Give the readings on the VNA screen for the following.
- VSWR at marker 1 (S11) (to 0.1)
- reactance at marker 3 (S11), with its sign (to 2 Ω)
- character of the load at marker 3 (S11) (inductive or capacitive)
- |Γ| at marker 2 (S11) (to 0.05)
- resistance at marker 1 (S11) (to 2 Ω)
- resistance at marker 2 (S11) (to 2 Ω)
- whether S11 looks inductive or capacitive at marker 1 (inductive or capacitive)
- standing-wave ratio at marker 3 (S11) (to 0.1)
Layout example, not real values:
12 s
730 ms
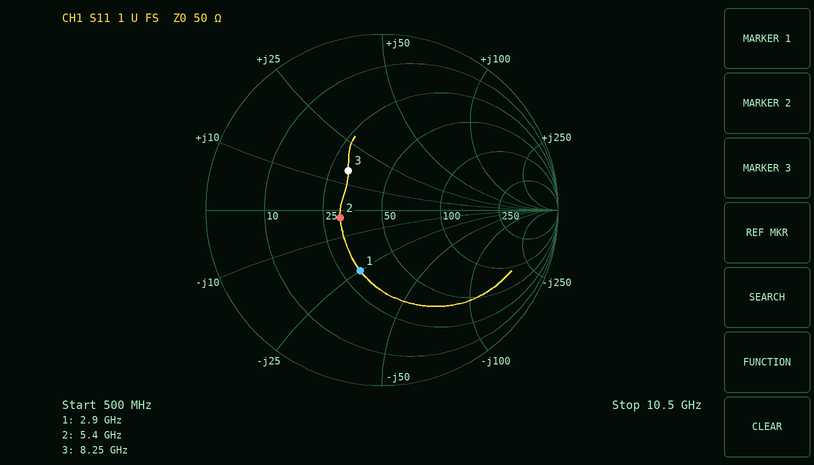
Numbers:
2.2
+16 Ω
inductive
0.25
32 Ω
30 Ω
capacitive
1.8
